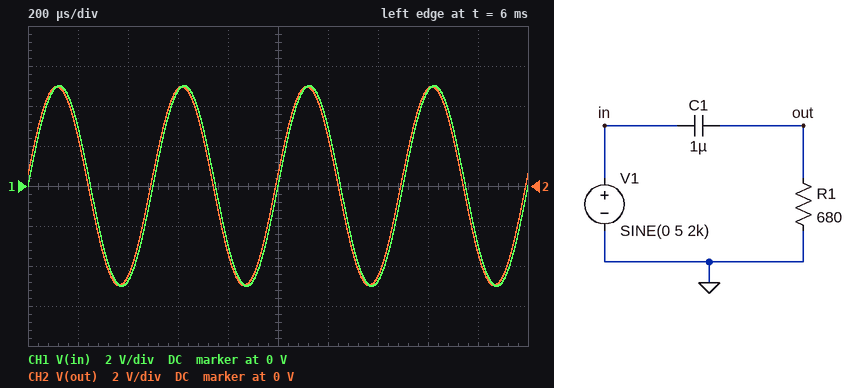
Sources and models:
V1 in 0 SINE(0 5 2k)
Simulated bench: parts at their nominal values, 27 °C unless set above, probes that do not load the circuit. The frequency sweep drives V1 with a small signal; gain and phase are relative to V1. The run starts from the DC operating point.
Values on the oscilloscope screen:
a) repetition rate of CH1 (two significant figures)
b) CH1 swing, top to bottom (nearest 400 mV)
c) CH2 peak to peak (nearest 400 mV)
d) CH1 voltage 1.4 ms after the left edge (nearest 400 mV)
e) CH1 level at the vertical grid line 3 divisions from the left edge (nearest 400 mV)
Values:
2.0 kHz
10.0 V
10.0 V
-4.8 V
4.8 V
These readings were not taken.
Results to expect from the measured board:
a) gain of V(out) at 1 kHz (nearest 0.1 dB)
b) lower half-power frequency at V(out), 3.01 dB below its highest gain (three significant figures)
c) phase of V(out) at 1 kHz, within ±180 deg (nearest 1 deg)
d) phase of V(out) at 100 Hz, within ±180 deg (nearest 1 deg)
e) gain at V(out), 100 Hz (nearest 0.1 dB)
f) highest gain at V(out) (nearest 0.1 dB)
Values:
-0.2 dB
234 Hz
13 deg
67 deg
-8.1 dB
0 dB
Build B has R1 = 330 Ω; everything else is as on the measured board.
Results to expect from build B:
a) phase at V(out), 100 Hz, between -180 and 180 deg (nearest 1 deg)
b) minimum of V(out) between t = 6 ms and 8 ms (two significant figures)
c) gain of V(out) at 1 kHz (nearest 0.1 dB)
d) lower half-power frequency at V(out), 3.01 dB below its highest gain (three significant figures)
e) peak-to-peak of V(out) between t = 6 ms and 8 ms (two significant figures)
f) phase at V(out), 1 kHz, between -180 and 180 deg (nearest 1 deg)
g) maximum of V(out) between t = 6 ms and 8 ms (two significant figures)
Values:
78 deg
-4.9 V
-0.9 dB
482 Hz
9.7 V
26 deg
4.9 V
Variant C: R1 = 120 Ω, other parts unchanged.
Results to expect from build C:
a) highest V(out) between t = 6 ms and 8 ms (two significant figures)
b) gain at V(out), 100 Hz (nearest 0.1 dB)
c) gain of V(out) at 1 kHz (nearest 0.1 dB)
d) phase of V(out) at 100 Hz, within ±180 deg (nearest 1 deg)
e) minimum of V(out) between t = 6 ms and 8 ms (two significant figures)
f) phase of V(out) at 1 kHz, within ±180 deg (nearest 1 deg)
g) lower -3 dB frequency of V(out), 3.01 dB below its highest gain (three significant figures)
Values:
4.2 V
-22.5 dB
-4.4 dB
86 deg
-4.2 V
53 deg
1.33 kHz
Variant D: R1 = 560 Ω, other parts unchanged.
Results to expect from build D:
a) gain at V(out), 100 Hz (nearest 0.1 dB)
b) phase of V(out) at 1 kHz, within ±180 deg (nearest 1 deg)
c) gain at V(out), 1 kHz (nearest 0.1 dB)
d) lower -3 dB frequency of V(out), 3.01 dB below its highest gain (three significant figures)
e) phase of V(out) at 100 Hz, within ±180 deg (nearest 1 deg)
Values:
-9.6 dB
16 deg
-0.3 dB
284 Hz
71 deg
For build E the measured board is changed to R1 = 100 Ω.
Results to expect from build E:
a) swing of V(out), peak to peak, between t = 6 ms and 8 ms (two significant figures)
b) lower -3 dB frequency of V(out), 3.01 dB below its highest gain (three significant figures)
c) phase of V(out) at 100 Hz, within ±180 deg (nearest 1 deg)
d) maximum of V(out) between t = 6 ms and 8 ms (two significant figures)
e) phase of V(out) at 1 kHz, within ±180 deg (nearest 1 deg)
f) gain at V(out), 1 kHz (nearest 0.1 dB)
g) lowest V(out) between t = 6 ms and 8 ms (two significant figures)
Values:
7.8 V
1.59 kHz
86 deg
3.9 V
58 deg
-5.5 dB
-3.9 V
